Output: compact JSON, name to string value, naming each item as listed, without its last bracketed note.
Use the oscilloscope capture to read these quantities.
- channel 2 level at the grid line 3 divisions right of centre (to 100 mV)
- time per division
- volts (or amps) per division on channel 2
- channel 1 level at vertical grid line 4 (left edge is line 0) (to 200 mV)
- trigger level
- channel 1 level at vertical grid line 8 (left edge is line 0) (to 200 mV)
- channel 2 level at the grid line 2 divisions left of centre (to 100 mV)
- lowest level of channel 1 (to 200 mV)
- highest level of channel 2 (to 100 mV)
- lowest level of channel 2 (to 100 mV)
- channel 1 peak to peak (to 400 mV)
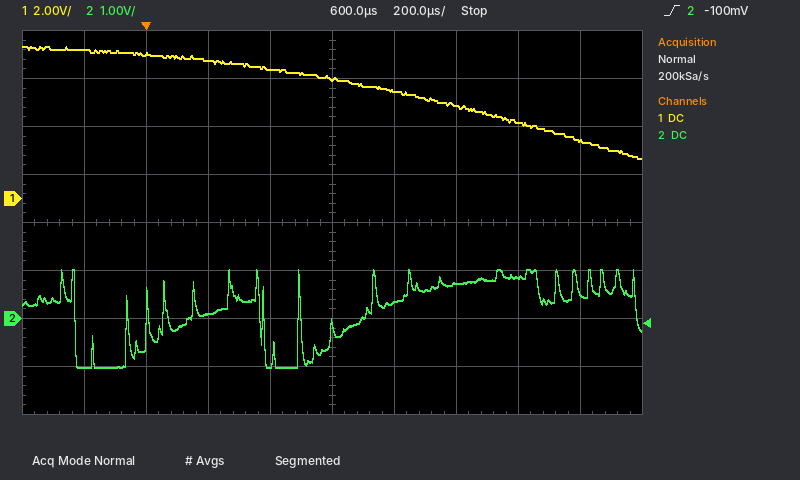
{"channel 2 level at the grid line 3 divisions right of centre": "900 mV", "time per division": "200 µs", "volts (or amps) per division on channel 2": "1 V", "channel 1 level at vertical grid line 4 (left edge is line 0)": "5.4 V", "trigger level": "-100 mV", "channel 1 level at vertical grid line 8 (left edge is line 0)": "3.2 V", "channel 2 level at the grid line 2 divisions left of centre": "100 mV", "lowest level of channel 1": "1.6 V", "highest level of channel 2": "1.0 V", "lowest level of channel 2": "-1.0 V", "channel 1 peak to peak": "4.8 V"}
